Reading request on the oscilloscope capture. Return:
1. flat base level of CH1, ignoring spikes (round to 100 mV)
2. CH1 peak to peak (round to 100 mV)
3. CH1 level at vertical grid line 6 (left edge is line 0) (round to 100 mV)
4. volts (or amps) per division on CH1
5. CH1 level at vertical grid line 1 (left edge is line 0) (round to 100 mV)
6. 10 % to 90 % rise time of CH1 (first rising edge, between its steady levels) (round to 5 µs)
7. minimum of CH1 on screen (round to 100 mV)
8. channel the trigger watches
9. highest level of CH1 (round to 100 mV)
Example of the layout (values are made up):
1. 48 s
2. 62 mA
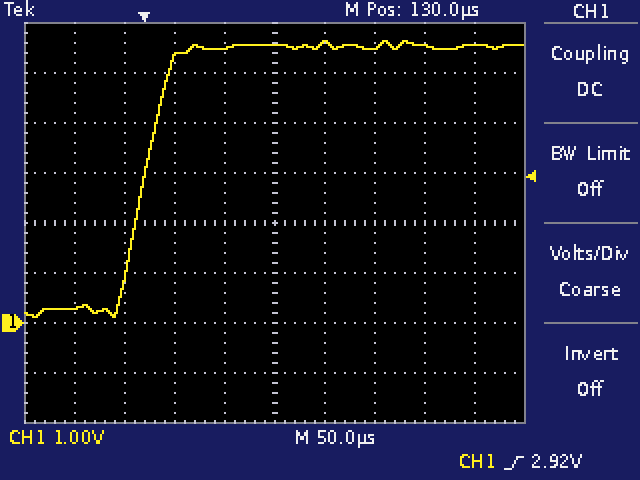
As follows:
1. 300 mV
2. 5.5 V
3. 5.6 V
4. 1 V
5. 300 mV
6. 45 µs
7. 100 mV
8. CH1
9. 5.6 V
